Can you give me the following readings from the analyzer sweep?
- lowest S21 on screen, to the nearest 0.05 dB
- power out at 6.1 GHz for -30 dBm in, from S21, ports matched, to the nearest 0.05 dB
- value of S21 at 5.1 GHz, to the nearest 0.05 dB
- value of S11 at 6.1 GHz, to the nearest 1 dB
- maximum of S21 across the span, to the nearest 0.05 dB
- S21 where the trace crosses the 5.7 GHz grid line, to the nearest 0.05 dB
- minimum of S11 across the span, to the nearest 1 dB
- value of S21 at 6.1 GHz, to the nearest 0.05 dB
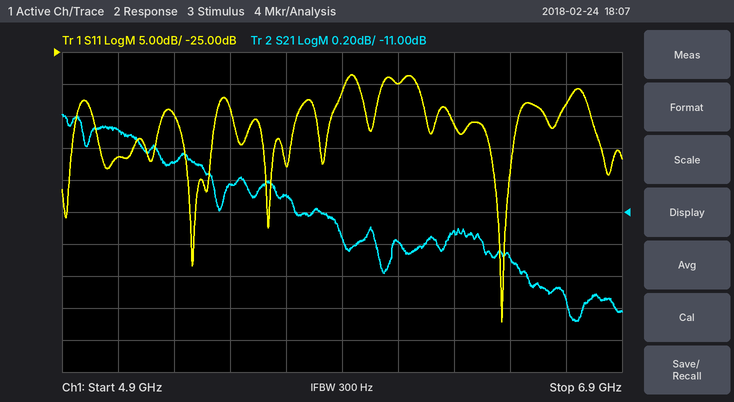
-11.70 dB
-41.20 dBm
-10.50 dB
-30 dB
-10.40 dB
-10.90 dB
-67 dB
-11.20 dB
